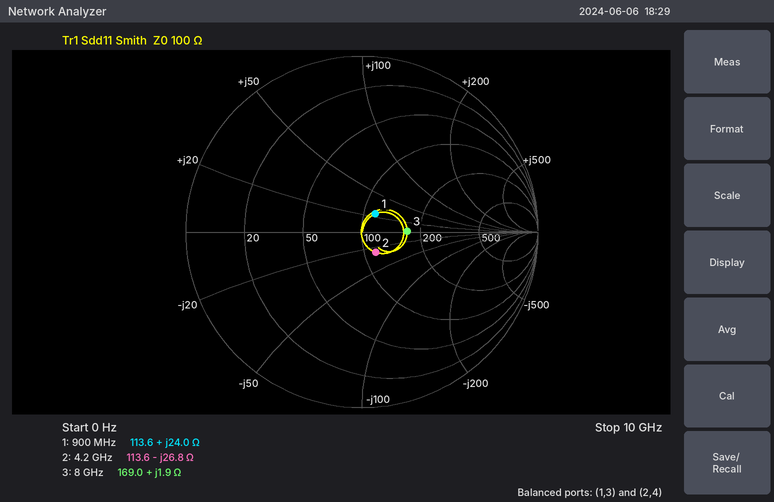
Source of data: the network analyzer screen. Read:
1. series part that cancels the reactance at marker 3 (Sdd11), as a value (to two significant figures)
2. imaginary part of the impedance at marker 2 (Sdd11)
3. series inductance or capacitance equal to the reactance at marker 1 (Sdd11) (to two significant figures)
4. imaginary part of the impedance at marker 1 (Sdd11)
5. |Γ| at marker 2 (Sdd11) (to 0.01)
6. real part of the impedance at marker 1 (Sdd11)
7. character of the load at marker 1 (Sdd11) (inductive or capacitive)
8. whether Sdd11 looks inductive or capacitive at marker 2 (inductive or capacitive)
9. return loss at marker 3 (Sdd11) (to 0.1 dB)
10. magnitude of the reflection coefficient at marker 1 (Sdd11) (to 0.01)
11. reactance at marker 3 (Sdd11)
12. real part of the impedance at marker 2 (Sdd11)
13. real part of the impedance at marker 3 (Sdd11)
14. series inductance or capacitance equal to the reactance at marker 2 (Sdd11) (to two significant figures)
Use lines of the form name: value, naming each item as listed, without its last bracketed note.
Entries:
series part that cancels the reactance at marker 3 (Sdd11), as a value: 10 pF
imaginary part of the impedance at marker 2: -26.8 Ω
series inductance or capacitance equal to the reactance at marker 1 (Sdd11): 4.2 nH
imaginary part of the impedance at marker 1: +24.0 Ω
|Γ| at marker 2 (Sdd11): 0.14
real part of the impedance at marker 1: 113.6 Ω
character of the load at marker 1 (Sdd11): inductive
whether Sdd11 looks inductive or capacitive at marker 2: capacitive
return loss at marker 3 (Sdd11): 11.8 dB
magnitude of the reflection coefficient at marker 1 (Sdd11): 0.13
reactance at marker 3: +1.9 Ω
real part of the impedance at marker 2: 113.6 Ω
real part of the impedance at marker 3: 169.0 Ω
series inductance or capacitance equal to the reactance at marker 2 (Sdd11): 1.4 pF
